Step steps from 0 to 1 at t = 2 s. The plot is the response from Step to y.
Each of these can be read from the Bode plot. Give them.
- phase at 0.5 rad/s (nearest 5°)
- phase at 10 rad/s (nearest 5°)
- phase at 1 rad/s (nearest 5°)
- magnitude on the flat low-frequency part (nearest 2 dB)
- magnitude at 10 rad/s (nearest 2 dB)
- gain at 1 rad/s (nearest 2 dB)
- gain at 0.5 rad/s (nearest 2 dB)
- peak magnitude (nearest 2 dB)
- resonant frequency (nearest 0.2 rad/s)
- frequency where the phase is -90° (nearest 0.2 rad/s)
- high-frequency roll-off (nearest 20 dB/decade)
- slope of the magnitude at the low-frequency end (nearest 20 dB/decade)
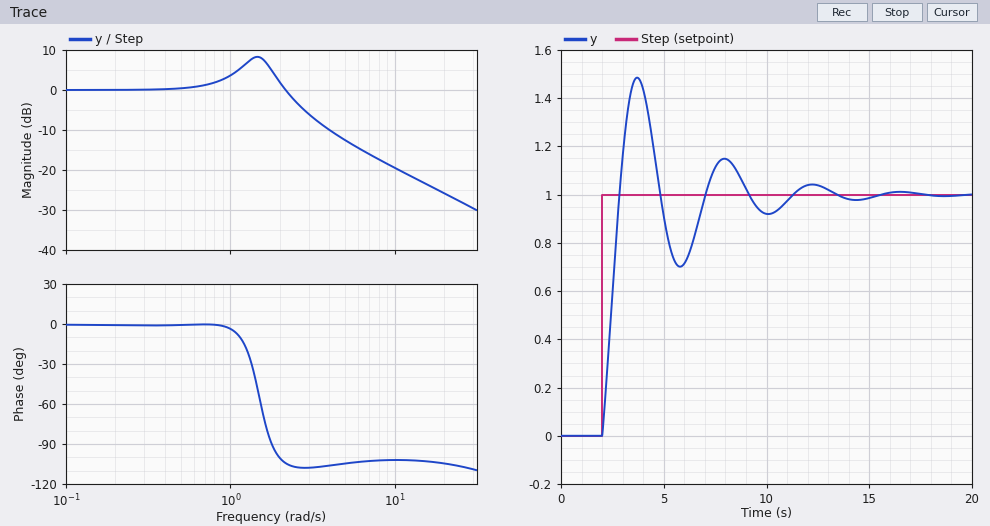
0°
-100°
-5°
0 dB
-20 dB
4 dB
0 dB
8 dB
1.4 rad/s
1.8 rad/s
-20 dB/decade
0 dB/decade
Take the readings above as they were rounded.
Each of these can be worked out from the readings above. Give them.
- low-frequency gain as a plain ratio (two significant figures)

1.0
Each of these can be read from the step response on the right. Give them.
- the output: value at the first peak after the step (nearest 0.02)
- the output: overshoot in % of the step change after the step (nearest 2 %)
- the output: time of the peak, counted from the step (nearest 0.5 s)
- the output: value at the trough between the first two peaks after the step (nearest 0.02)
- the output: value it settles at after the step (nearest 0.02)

1.48
48 %
1.5 s
0.70
1.00
